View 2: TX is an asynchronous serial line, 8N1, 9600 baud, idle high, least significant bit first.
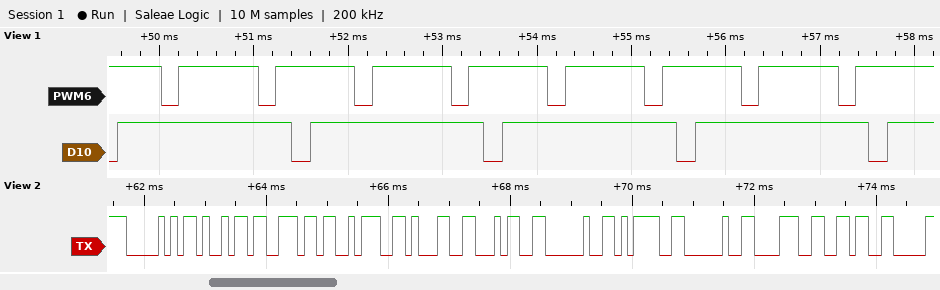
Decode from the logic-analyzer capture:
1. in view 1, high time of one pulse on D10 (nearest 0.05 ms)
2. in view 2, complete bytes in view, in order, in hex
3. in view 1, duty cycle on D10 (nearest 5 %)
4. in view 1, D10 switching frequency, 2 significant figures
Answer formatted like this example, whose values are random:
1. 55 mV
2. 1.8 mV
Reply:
1. 1.85 ms
2. 50 69 6E 3A 31 34 20 3D 20 38 36
3. 90 %
4. 490 Hz
